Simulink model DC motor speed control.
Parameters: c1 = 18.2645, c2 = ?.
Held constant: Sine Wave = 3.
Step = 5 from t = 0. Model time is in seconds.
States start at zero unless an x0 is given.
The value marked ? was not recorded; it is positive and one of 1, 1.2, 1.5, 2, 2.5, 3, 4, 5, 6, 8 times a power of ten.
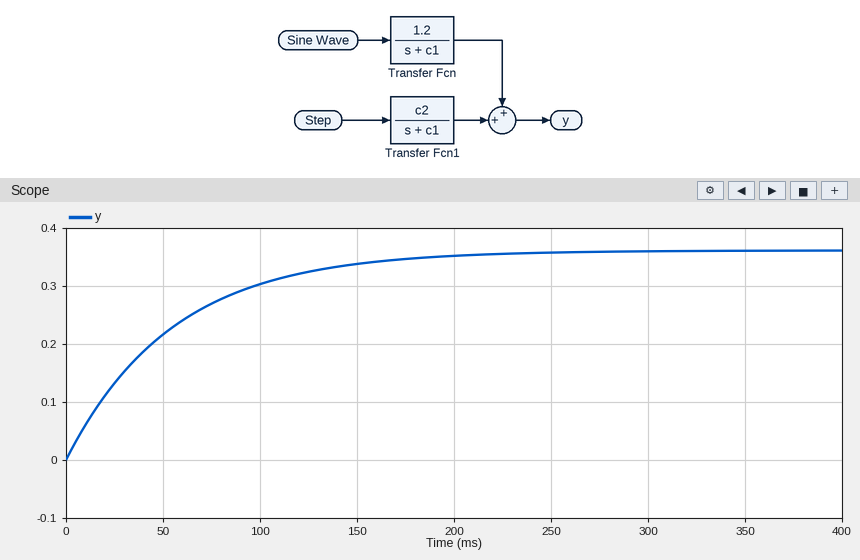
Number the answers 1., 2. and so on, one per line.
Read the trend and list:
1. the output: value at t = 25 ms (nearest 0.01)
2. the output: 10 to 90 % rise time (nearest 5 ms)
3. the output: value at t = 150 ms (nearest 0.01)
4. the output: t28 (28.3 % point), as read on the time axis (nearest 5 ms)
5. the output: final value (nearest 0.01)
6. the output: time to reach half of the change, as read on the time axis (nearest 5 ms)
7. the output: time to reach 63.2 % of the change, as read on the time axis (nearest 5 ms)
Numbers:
1. 0.13
2. 120 ms
3. 0.34
4. 20 ms
5. 0.36
6. 40 ms
7. 55 ms
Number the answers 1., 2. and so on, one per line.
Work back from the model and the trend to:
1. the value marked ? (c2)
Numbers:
1. 0.6
